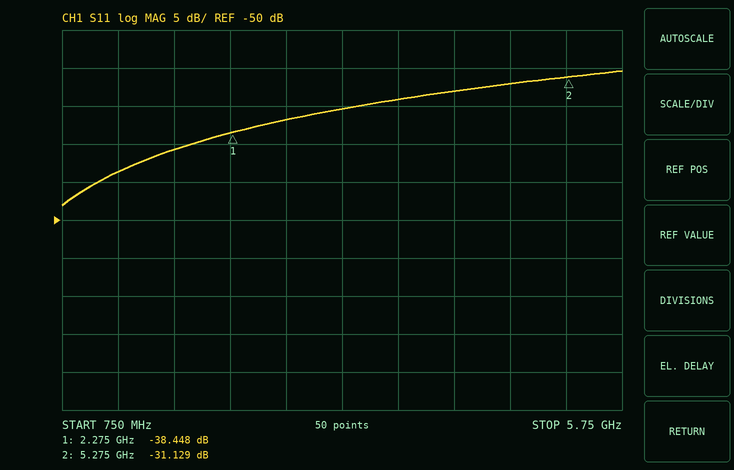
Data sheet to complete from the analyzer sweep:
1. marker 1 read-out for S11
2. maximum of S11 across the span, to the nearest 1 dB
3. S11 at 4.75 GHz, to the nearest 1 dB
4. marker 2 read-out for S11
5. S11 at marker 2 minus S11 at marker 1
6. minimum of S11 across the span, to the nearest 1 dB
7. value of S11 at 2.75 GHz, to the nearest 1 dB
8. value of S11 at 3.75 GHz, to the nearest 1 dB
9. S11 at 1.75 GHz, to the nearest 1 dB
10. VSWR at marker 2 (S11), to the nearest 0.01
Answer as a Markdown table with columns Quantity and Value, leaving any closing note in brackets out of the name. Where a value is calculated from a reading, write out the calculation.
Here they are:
| Quantity | Value |
|---|---|
| marker 1 read-out for S11 | -38.448 dB |
| maximum of S11 across the span, to the nearest 1 dB | -30 dB |
| S11 at 4.75 GHz, to the nearest 1 dB | -32 dB |
| marker 2 read-out for S11 | -31.129 dB |
| S11 at marker 2 minus S11 at marker 1 | -31.129 − (-38.448) = 7.319 dB |
| minimum of S11 across the span, to the nearest 1 dB | -48 dB |
| value of S11 at 2.75 GHz, to the nearest 1 dB | -37 dB |
| value of S11 at 3.75 GHz, to the nearest 1 dB | -34 dB |
| S11 at 1.75 GHz, to the nearest 1 dB | -41 dB |
| VSWR at marker 2 (S11), to the nearest 0.01 | (1 + 0.0278)/(1 − 0.0278) ≈ 1.06 |
